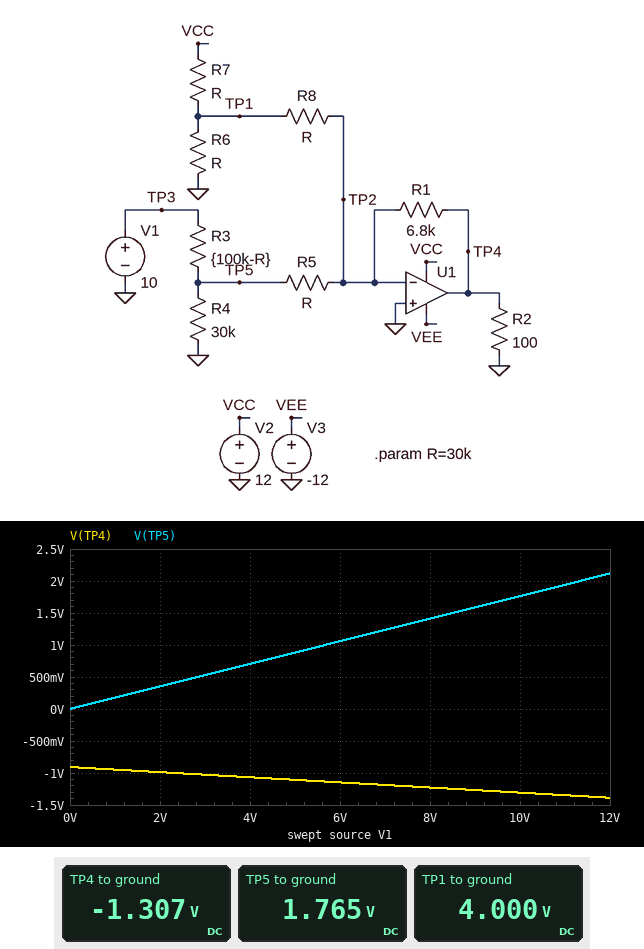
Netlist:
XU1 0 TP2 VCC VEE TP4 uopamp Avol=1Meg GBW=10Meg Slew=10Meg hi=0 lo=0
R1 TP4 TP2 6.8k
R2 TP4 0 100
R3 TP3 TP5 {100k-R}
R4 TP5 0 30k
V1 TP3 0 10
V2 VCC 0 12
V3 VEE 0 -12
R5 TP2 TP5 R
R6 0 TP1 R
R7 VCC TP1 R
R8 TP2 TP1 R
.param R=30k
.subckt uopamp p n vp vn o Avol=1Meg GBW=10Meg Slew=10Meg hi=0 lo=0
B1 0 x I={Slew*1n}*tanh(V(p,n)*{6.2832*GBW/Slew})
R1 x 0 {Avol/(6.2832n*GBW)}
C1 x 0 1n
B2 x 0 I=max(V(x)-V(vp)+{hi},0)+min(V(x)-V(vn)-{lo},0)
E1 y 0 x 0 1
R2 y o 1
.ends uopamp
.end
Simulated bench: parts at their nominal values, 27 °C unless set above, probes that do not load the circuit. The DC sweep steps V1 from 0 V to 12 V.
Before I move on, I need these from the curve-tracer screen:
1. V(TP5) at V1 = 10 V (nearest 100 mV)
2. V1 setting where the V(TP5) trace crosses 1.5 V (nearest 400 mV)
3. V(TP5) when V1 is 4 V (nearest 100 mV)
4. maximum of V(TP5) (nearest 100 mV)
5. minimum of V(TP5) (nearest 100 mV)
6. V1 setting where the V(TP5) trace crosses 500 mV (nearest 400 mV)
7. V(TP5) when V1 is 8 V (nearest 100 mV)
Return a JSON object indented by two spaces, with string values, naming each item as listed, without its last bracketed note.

{
  "V(TP5) at V1 = 10 V": "1.8 V",
  "V1 setting where the V(TP5) trace crosses 1.5 V": "8.4 V",
  "V(TP5) when V1 is 4 V": "700 mV",
  "maximum of V(TP5)": "2.1 V",
  "minimum of V(TP5)": "0 V",
  "V1 setting where the V(TP5) trace crosses 500 mV": "2.8 V",
  "V(TP5) when V1 is 8 V": "1.4 V"
}
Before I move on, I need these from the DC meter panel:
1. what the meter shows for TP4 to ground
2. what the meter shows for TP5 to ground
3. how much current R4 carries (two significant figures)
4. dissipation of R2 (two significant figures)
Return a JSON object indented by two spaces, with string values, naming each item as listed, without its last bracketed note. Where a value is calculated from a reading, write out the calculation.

{
  "what the meter shows for TP4 to ground": "-1.307 V",
  "what the meter shows for TP5 to ground": "1.765 V",
  "how much current R4 carries": "(1.765 V) / 30 kΩ = 59 µA",
  "dissipation of R2": "(0 V - (-1.307 V))^2 / 100 Ω = 17 mW"
}
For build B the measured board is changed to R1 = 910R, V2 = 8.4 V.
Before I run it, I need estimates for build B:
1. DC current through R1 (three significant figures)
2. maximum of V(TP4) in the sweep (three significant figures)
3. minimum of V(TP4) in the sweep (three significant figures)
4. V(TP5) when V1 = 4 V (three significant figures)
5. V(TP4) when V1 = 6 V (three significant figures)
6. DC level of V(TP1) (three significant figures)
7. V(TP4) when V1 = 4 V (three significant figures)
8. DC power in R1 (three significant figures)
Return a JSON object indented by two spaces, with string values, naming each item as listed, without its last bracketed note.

{
  "DC current through R1": "152 µA",
  "maximum of V(TP4) in the sweep": "-84.9 mV",
  "minimum of V(TP4) in the sweep": "-149 mV",
  "V(TP5) when V1 = 4 V": "706 mV",
  "V(TP4) when V1 = 6 V": "-117 mV",
  "DC level of V(TP1)": "2.80 V",
  "V(TP4) when V1 = 4 V": "-106 mV",
  "DC power in R1": "21.1 µW"
}
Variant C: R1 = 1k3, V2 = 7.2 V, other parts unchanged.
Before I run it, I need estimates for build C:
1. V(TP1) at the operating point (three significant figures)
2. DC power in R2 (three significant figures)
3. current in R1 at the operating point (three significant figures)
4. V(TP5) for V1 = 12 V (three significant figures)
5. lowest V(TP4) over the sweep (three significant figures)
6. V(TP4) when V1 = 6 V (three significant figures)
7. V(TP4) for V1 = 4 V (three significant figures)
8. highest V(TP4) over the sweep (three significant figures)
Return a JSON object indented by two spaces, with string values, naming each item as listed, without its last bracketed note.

{
  "V(TP1) at the operating point": "2.40 V",
  "DC power in R2": "326 µW",
  "current in R1 at the operating point": "139 µA",
  "V(TP5) for V1 = 12 V": "2.12 V",
  "lowest V(TP4) over the sweep": "-196 mV",
  "V(TP4) when V1 = 6 V": "-150 mV",
  "V(TP4) for V1 = 4 V": "-135 mV",
  "highest V(TP4) over the sweep": "-104 mV"
}
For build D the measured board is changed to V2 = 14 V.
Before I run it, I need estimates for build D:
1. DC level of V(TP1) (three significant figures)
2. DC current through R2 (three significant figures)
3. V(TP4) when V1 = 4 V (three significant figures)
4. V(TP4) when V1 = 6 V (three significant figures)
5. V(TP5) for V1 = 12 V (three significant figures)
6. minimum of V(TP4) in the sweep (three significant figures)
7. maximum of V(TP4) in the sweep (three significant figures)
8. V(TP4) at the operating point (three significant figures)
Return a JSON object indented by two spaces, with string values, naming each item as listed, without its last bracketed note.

{
  "DC level of V(TP1)": "4.67 V",
  "DC current through R2": "14.6 mA",
  "V(TP4) when V1 = 4 V": "-1.22 V",
  "V(TP4) when V1 = 6 V": "-1.30 V",
  "V(TP5) for V1 = 12 V": "2.12 V",
  "minimum of V(TP4) in the sweep": "-1.54 V",
  "maximum of V(TP4) in the sweep": "-1.06 V",
  "V(TP4) at the operating point": "-1.46 V"
}
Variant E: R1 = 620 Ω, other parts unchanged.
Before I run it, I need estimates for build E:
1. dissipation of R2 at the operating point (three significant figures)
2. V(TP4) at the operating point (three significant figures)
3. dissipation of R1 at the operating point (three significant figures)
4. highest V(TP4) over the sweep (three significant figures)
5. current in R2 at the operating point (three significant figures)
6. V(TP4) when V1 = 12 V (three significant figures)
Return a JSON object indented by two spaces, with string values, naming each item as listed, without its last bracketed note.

{
  "dissipation of R2 at the operating point": "142 µW",
  "V(TP4) at the operating point": "-119 mV",
  "dissipation of R1 at the operating point": "22.9 µW",
  "highest V(TP4) over the sweep": "-82.7 mV",
  "current in R2 at the operating point": "1.19 mA",
  "V(TP4) when V1 = 12 V": "-126 mV"
}
